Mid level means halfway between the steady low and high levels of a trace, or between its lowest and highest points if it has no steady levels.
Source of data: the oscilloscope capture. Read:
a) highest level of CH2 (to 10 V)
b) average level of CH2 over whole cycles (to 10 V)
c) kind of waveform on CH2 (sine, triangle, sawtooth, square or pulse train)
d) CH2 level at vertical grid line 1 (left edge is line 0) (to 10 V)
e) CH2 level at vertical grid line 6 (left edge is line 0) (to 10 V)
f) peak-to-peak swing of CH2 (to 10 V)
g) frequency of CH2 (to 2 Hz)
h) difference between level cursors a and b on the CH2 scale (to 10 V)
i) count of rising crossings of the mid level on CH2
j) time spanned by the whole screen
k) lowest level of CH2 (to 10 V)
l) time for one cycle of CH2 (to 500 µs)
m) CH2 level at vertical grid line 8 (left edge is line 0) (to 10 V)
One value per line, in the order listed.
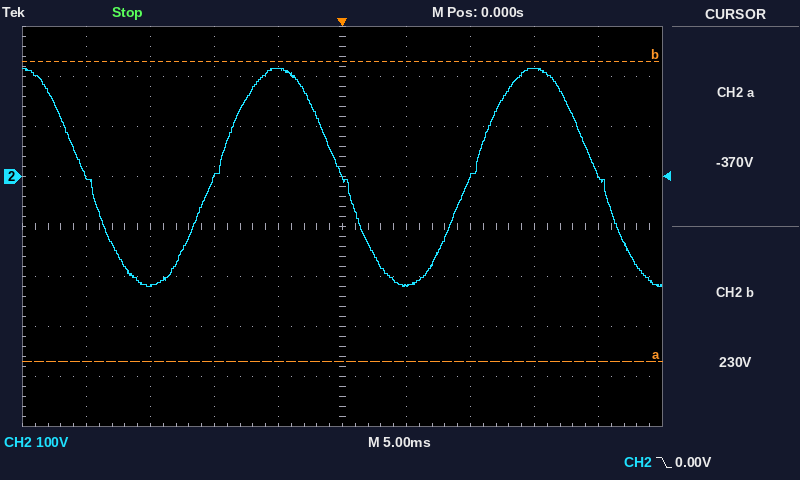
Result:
220 V
0 V
sine
0 V
-220 V
440 V
50 Hz
600 V
2
50 ms
-220 V
20.0 ms
220 V
